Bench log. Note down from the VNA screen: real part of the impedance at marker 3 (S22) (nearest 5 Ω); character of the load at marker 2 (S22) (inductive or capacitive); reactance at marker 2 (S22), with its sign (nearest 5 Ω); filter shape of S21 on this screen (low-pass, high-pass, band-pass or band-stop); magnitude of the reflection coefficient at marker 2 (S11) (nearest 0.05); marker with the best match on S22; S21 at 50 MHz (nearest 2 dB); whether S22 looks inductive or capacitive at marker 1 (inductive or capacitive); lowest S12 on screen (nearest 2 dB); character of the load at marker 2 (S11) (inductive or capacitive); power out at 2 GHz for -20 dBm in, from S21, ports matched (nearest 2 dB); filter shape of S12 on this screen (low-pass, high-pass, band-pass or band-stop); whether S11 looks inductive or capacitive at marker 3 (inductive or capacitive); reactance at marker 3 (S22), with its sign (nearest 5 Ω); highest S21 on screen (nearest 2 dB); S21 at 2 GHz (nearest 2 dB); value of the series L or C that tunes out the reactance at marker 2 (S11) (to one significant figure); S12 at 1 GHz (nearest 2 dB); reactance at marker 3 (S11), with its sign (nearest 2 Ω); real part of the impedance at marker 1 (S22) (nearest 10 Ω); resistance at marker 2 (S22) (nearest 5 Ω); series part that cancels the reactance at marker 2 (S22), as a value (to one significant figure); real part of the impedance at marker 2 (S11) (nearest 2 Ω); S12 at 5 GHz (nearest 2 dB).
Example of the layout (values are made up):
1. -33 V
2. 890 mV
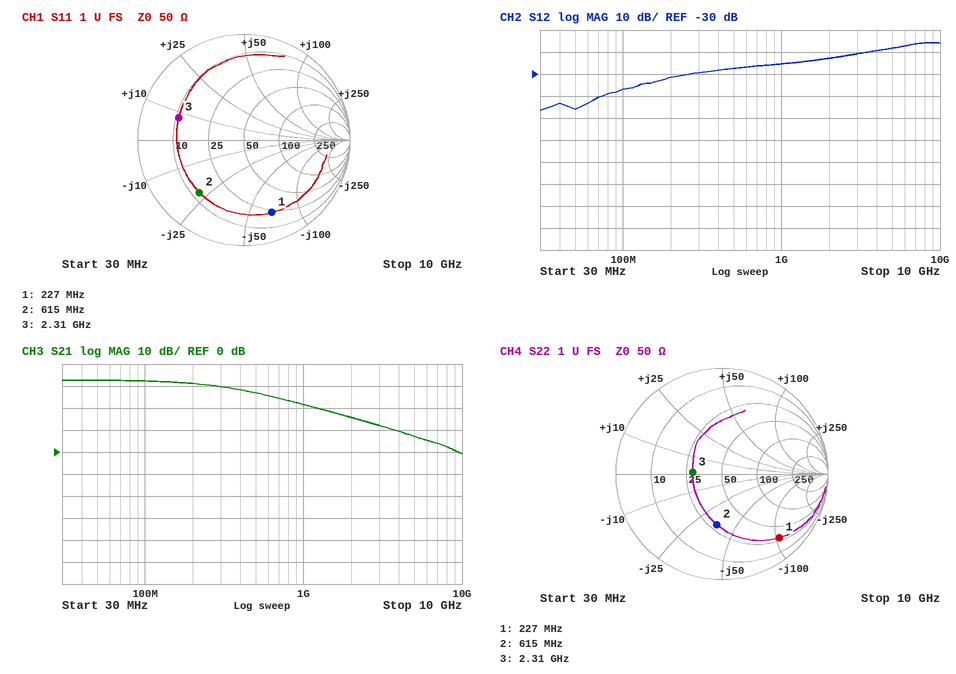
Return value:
1. 30 Ω
2. capacitive
3. -35 Ω
4. low-pass
5. 0.65
6. marker 3
7. 32 dB
8. capacitive
9. -46 dB
10. capacitive
11. -4 dBm
12. high-pass
13. inductive
14. 0 Ω
15. 32 dB
16. 16 dB
17. 6 nH
18. -26 dB
19. +8 Ω
20. 30 Ω
21. 30 Ω
22. 9 nH
23. 12 Ω
24. -18 dB
